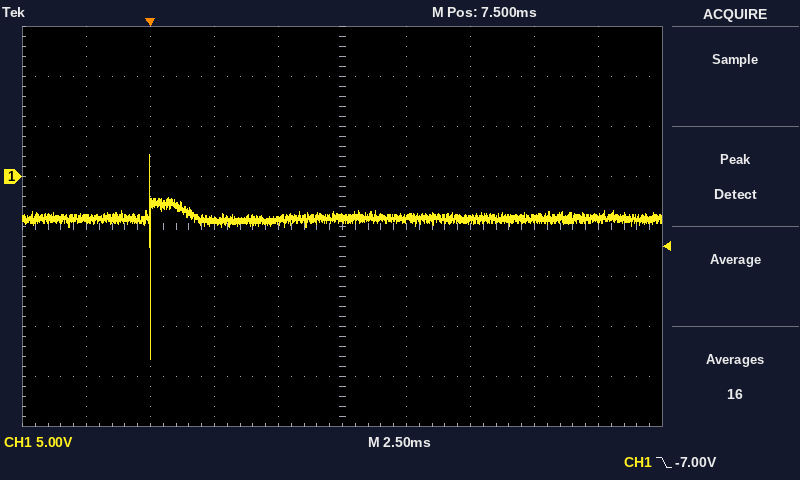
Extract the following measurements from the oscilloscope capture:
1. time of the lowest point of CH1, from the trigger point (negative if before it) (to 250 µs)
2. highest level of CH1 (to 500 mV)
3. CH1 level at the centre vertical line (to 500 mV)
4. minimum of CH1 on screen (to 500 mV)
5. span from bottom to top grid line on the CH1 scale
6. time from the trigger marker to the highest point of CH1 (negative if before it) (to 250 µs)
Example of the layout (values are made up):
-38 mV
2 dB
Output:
0.00 ms
2.0 V
-4.0 V
-18.0 V
40 V
0.00 ms
